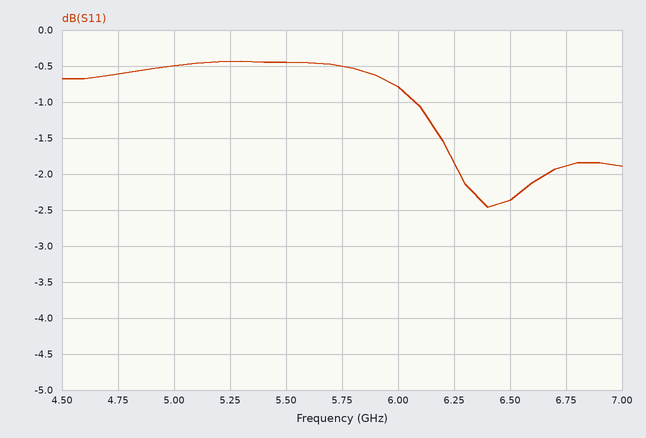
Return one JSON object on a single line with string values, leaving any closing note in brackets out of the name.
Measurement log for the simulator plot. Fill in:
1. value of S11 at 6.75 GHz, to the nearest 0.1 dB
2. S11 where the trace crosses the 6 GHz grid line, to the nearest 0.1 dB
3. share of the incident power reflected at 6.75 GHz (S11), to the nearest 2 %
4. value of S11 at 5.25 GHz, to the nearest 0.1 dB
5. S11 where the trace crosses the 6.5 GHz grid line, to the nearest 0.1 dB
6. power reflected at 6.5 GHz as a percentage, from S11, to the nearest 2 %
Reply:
{"value of S11 at 6.75 GHz, to the nearest 0.1 dB": "-1.9 dB", "S11 where the trace crosses the 6 GHz grid line, to the nearest 0.1 dB": "-0.8 dB", "share of the incident power reflected at 6.75 GHz (S11), to the nearest 2 %": "64 %", "value of S11 at 5.25 GHz, to the nearest 0.1 dB": "-0.4 dB", "S11 where the trace crosses the 6.5 GHz grid line, to the nearest 0.1 dB": "-2.4 dB", "power reflected at 6.5 GHz as a percentage, from S11, to the nearest 2 %": "58 %"}
